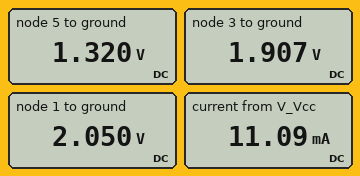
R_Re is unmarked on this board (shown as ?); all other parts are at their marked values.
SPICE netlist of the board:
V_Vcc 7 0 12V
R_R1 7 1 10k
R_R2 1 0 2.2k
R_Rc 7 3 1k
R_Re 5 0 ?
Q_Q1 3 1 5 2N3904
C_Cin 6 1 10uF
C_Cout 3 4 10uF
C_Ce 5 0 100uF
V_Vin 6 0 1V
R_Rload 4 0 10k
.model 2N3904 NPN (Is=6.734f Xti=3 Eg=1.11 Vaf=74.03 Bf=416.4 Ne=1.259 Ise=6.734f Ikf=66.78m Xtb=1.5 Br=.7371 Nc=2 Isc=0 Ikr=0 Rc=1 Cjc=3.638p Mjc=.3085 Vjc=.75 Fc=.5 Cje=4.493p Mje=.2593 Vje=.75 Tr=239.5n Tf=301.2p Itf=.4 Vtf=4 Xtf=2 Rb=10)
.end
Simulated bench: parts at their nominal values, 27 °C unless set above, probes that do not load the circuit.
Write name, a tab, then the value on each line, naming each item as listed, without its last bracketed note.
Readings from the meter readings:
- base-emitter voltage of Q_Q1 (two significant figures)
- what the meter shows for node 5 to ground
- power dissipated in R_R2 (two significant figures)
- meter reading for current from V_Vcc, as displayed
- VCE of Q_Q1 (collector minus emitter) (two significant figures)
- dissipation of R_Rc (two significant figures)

base-emitter voltage of Q_Q1	730 mV
what the meter shows for node 5 to ground	1.320 V
power dissipated in R_R2	1.9 mW
meter reading for current from V_Vcc, as displayed	11.09 mA
VCE of Q_Q1 (collector minus emitter)	590 mV
dissipation of R_Rc	100 mW
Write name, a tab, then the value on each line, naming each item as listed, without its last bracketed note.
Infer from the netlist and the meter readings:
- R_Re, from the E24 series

R_Re, from the E24 series	130 Ω
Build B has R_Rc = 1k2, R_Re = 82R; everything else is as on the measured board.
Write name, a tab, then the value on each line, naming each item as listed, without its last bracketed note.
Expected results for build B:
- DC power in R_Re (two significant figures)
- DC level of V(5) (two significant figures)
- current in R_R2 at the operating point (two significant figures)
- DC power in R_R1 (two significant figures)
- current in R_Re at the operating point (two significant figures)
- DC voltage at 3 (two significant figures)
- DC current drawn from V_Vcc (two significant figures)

DC power in R_Re	7.6 mW
DC level of V(5)	790 mV
current in R_R2 at the operating point	690 µA
DC power in R_R1	11 mW
current in R_Re at the operating point	9.6 mA
DC voltage at 3	900 mV
DC current drawn from V_Vcc	10 mA
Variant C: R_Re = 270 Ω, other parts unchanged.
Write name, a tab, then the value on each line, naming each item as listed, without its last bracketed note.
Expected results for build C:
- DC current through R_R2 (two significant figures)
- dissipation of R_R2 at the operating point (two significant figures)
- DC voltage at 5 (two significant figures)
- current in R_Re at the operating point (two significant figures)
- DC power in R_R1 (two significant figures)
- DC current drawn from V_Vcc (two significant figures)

DC current through R_R2	960 µA
dissipation of R_R2 at the operating point	2.0 mW
DC voltage at 5	1.4 V
current in R_Re at the operating point	5.2 mA
DC power in R_R1	9.8 mW
DC current drawn from V_Vcc	6.1 mA
